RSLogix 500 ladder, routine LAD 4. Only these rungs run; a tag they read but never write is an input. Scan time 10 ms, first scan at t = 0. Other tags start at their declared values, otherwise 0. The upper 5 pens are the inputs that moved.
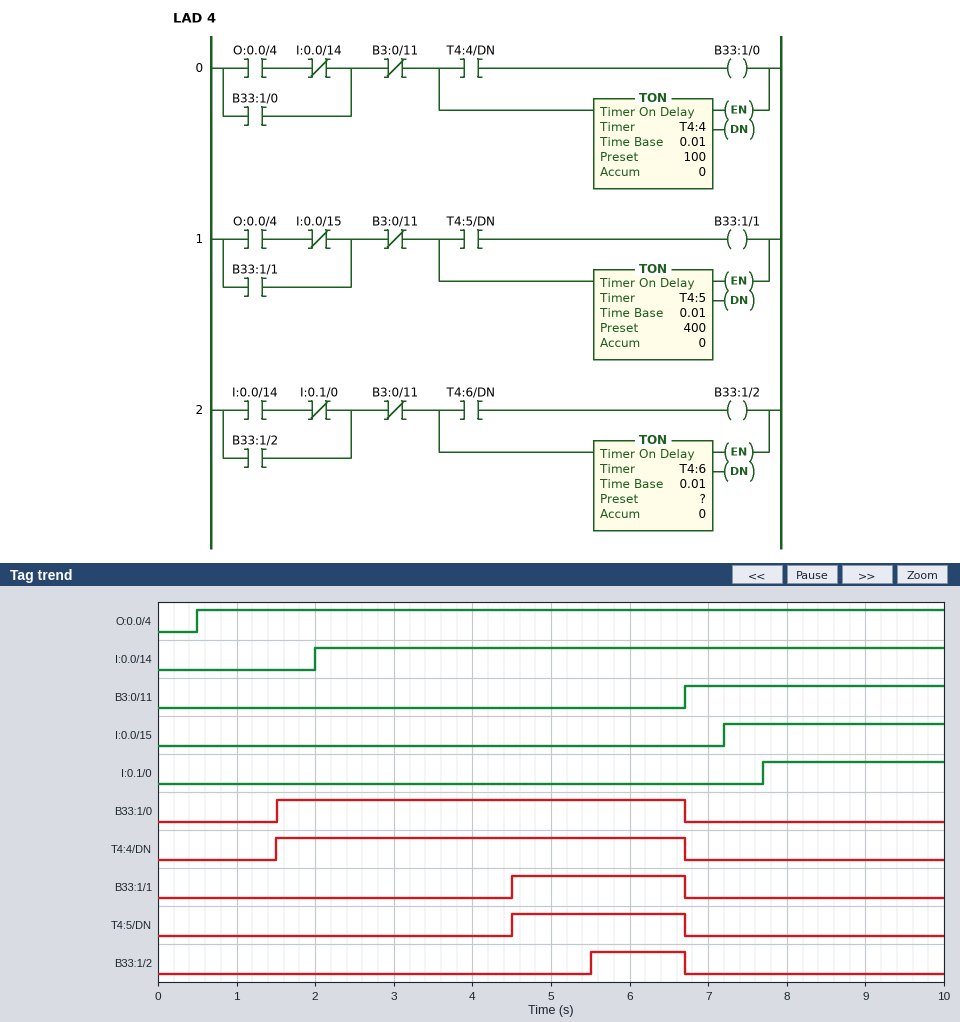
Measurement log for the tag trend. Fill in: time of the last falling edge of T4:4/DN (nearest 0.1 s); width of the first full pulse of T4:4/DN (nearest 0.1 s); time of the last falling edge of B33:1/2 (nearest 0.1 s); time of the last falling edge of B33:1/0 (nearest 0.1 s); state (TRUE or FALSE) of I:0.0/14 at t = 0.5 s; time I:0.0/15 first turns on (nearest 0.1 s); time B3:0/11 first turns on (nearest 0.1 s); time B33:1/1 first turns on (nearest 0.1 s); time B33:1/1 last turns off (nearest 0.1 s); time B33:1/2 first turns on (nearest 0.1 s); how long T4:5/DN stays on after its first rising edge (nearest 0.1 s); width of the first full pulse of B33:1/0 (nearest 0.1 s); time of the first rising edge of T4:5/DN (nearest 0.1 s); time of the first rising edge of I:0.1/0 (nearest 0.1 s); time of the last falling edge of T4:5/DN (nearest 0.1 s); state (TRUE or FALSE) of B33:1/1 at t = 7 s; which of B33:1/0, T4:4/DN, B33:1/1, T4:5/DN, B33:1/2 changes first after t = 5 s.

6.7 s
5.2 s
6.7 s
6.7 s
FALSE
7.2 s
6.7 s
4.5 s
6.7 s
5.5 s
2.2 s
5.2 s
4.5 s
7.7 s
6.7 s
FALSE
B33:1/2
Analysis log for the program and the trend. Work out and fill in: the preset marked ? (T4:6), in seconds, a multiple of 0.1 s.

3.5 s
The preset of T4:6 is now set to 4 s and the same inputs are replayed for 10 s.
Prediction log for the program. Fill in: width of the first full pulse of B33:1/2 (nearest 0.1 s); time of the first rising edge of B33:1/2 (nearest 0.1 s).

0.7 s
6.0 s
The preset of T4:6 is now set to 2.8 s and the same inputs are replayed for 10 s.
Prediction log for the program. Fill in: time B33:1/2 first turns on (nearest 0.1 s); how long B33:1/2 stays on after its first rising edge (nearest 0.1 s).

4.8 s
1.9 s
